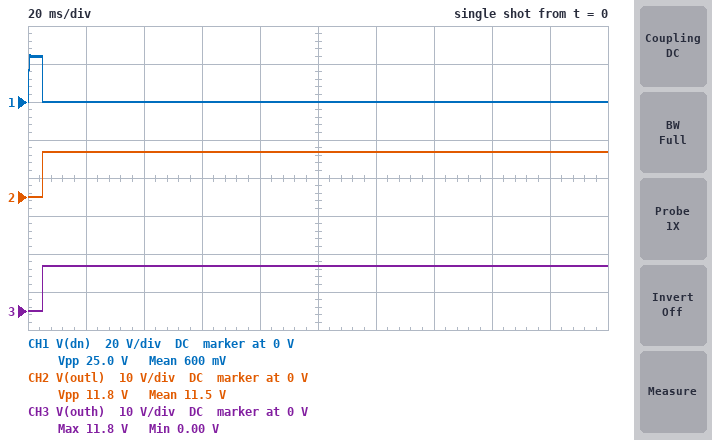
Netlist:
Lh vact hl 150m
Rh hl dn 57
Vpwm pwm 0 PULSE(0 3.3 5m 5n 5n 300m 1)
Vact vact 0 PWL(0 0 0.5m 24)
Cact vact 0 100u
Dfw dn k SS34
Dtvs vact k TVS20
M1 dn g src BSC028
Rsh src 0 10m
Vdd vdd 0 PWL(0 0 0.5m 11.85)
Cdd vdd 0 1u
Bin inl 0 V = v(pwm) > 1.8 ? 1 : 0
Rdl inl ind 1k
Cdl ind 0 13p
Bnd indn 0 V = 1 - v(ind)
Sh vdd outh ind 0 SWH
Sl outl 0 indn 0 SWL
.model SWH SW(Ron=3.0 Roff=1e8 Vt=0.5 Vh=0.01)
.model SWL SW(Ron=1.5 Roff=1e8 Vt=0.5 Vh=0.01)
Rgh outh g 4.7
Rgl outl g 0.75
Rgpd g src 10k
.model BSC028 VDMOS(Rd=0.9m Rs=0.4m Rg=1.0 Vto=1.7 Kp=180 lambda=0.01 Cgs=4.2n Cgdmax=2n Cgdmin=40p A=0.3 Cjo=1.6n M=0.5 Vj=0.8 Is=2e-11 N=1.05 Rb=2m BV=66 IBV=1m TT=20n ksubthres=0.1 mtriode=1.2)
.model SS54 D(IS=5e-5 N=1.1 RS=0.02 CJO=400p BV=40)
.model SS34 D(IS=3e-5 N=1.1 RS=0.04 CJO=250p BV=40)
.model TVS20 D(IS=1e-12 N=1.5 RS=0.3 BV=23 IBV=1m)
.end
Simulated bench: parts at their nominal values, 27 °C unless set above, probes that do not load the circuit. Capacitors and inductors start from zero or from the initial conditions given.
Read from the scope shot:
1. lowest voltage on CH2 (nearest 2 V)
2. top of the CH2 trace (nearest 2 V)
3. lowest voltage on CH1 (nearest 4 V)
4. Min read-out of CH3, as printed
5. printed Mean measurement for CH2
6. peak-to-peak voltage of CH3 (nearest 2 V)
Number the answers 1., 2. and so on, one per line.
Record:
1. 0 V
2. 12 V
3. 0 V
4. 0.00 V
5. 11.5 V
6. 12 V
